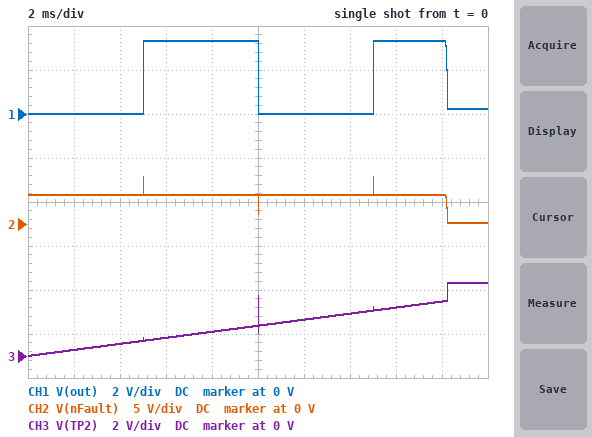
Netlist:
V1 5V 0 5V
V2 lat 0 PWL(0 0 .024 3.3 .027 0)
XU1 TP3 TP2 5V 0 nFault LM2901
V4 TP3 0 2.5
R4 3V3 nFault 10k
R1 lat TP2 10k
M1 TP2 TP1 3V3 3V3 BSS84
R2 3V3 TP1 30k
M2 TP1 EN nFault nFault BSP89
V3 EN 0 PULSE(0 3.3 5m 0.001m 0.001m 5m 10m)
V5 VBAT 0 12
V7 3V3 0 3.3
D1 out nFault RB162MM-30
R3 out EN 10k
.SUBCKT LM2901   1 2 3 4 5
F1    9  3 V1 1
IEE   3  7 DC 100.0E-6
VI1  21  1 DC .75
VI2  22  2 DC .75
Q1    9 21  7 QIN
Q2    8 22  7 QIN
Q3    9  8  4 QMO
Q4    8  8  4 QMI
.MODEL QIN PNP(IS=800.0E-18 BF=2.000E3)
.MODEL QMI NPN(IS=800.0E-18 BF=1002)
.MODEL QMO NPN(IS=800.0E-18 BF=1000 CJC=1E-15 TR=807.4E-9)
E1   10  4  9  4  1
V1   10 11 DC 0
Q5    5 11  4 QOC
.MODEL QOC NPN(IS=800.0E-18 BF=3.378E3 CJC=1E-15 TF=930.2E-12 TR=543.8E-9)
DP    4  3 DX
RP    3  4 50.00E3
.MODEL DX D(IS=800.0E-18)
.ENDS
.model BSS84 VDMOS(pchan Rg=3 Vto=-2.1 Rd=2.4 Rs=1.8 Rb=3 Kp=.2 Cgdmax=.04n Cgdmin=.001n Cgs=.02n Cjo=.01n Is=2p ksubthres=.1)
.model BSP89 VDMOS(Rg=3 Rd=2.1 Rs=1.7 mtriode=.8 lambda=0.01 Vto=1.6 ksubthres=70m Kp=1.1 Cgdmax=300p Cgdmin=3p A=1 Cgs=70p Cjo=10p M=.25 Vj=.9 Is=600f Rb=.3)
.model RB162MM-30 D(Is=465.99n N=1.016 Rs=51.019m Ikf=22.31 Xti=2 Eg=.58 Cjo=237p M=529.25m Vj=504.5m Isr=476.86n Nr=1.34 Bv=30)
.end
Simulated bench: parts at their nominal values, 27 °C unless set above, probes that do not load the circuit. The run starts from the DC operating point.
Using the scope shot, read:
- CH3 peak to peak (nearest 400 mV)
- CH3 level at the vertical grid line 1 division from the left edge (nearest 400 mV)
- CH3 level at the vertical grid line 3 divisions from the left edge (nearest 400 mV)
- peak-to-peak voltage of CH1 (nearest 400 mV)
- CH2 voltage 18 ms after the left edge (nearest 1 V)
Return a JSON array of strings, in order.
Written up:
["3.2 V", "400 mV", "800 mV", "3.2 V", "3 V"]
